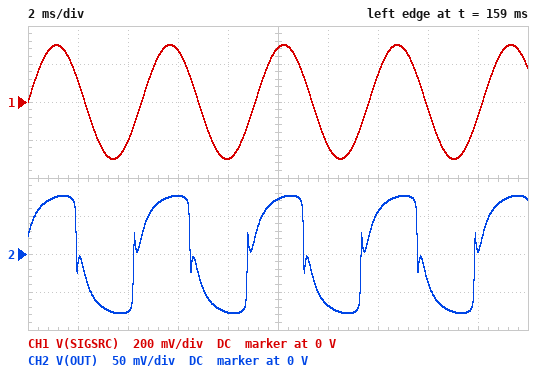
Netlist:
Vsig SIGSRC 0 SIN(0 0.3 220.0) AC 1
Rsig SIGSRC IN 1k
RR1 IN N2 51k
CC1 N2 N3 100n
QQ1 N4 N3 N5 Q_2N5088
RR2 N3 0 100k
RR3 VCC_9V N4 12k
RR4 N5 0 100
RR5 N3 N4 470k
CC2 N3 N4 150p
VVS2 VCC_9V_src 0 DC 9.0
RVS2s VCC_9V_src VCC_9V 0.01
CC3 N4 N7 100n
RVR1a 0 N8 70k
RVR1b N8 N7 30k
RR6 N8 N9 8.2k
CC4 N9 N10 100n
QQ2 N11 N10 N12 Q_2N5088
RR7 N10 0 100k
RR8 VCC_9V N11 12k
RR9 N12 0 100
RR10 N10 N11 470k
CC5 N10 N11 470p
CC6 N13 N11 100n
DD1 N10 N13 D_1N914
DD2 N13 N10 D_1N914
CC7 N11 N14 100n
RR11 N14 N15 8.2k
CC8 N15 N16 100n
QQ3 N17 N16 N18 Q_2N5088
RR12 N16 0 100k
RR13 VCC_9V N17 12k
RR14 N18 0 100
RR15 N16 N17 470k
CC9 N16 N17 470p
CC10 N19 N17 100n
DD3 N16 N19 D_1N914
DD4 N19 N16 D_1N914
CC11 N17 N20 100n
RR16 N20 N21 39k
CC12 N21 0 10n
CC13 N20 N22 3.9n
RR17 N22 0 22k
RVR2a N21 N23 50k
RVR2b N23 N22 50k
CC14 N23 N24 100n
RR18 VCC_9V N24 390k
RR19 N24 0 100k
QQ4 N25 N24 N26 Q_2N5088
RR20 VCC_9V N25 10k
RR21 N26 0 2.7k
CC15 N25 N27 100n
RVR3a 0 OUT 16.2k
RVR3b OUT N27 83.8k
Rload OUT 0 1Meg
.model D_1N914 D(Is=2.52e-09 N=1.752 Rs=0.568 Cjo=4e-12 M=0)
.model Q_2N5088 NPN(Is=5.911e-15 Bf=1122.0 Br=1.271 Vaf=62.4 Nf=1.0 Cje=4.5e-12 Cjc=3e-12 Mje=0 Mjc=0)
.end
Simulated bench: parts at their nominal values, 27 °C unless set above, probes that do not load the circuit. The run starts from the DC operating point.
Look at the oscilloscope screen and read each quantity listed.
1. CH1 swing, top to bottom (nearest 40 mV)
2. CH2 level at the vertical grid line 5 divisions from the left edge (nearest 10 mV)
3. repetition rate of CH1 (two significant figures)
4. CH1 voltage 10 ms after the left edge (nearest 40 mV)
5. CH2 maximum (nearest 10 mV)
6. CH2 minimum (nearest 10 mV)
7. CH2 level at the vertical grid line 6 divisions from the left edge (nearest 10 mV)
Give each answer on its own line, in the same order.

600 mV
70 mV
220 Hz
280 mV
80 mV
-80 mV
-70 mV
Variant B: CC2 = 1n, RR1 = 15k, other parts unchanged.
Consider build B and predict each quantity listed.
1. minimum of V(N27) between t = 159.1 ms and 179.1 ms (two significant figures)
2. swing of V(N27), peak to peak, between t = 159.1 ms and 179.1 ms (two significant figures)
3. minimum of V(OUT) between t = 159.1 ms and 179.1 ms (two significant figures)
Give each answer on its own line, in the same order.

-580 mV
1.2 V
-92 mV
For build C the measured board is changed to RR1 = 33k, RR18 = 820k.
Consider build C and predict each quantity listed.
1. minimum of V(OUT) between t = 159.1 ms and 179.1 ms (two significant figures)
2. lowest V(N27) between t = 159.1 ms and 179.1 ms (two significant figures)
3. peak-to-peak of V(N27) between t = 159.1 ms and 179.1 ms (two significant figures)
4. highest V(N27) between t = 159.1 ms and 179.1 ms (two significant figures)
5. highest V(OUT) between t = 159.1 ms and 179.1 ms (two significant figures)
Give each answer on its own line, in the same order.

-83 mV
-520 mV
1.0 V
510 mV
82 mV
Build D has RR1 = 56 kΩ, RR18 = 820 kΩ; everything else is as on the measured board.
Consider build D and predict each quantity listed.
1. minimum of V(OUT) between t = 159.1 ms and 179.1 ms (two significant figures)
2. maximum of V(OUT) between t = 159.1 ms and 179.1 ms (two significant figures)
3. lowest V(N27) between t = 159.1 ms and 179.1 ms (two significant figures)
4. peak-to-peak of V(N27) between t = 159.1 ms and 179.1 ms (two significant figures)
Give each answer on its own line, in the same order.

-77 mV
74 mV
-480 mV
940 mV
